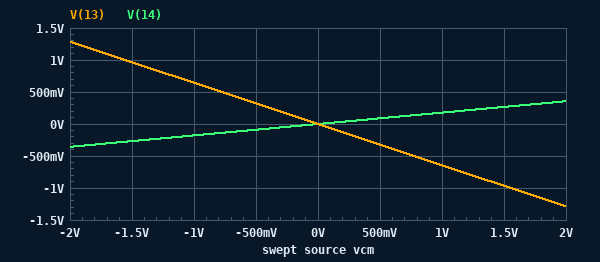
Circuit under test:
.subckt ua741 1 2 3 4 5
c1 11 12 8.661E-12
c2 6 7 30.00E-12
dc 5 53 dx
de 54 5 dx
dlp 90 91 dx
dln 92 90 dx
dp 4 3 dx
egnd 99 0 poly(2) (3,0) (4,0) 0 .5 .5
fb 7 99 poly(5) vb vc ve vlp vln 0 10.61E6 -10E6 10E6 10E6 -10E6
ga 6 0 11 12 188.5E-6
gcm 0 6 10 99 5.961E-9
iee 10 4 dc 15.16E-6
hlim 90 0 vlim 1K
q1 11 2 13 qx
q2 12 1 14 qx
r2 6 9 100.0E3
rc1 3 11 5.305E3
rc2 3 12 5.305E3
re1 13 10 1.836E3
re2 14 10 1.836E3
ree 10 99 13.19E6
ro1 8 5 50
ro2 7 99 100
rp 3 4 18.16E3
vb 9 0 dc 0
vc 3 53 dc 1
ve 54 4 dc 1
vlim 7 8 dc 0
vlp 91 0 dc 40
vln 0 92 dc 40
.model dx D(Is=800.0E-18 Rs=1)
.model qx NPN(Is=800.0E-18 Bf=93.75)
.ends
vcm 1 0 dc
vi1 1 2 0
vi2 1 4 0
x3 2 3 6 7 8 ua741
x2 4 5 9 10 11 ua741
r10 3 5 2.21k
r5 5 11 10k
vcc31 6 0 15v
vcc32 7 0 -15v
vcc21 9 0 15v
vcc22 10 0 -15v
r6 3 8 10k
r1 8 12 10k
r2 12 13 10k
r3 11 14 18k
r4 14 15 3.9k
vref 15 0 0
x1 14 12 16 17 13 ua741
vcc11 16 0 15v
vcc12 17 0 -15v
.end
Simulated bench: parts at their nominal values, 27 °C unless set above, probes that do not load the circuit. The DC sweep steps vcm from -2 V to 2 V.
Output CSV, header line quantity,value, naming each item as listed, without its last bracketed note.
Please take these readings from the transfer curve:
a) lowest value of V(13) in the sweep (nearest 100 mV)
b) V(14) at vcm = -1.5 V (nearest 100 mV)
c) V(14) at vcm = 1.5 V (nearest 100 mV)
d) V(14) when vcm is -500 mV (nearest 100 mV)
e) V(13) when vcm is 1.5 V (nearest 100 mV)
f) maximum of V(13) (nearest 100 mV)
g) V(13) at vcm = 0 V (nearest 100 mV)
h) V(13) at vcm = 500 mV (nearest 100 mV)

quantity,value
lowest value of V(13) in the sweep,-1.3 V
V(14) at vcm = -1.5 V,-300 mV
V(14) at vcm = 1.5 V,300 mV
V(14) when vcm is -500 mV,-100 mV
V(13) when vcm is 1.5 V,-1.0 V
maximum of V(13),1.3 V
V(13) at vcm = 0 V,0 V
V(13) at vcm = 500 mV,-300 mV
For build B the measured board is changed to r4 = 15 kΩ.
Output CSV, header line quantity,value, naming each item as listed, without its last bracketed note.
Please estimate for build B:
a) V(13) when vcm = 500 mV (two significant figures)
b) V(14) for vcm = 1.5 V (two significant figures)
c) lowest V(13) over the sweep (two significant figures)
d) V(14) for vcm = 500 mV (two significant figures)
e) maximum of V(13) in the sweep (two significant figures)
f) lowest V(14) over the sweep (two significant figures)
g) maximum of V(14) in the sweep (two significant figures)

quantity,value
V(13) when vcm = 500 mV,-46 mV
V(14) for vcm = 1.5 V,680 mV
lowest V(13) over the sweep,-180 mV
V(14) for vcm = 500 mV,230 mV
maximum of V(13) in the sweep,180 mV
lowest V(14) over the sweep,-910 mV
maximum of V(14) in the sweep,910 mV
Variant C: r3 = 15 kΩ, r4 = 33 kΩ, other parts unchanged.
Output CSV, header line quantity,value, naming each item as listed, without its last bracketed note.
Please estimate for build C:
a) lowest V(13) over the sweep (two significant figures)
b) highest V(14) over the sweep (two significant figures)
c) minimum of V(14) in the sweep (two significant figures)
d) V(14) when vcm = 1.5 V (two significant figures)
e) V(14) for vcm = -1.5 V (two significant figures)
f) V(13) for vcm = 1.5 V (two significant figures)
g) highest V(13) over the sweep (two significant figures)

quantity,value
lowest V(13) over the sweep,-750 mV
highest V(14) over the sweep,1.4 V
minimum of V(14) in the sweep,-1.4 V
V(14) when vcm = 1.5 V,1.0 V
V(14) for vcm = -1.5 V,-1.0 V
V(13) for vcm = 1.5 V,560 mV
highest V(13) over the sweep,750 mV
